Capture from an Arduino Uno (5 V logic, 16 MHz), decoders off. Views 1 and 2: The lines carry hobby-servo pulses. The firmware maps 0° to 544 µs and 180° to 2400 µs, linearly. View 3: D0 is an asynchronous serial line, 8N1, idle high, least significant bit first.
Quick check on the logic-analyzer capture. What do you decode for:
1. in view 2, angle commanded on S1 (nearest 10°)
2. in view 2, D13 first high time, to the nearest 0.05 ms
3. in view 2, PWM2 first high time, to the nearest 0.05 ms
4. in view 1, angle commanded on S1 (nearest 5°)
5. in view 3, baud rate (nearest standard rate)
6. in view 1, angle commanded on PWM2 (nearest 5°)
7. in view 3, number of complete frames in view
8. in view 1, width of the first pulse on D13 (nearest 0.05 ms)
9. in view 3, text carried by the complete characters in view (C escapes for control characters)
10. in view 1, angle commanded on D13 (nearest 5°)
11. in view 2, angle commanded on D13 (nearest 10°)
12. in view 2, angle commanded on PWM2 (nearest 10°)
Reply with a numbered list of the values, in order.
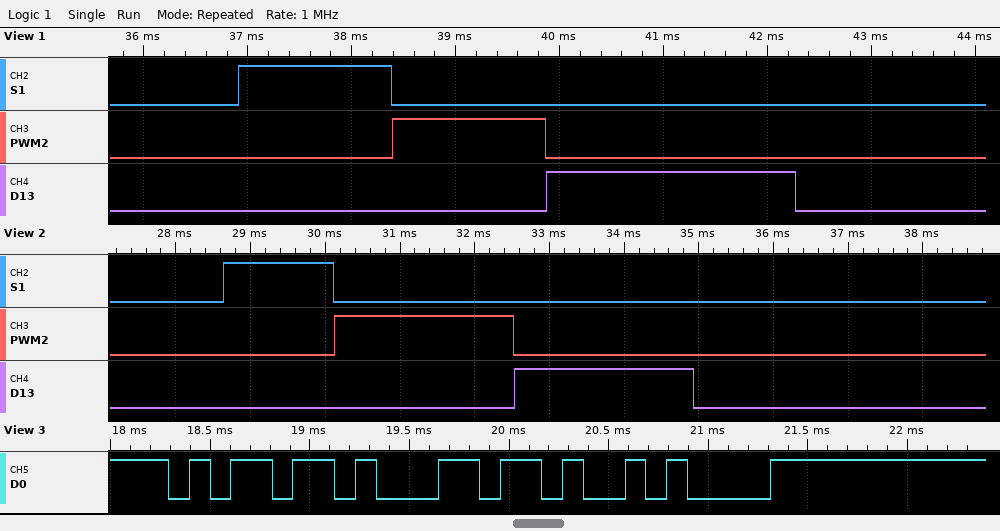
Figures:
1. 90°
2. 2.40 ms
3. 2.40 ms
4. 90°
5. 9600 baud
6. 90°
7. 3
8. 2.40 ms
9. "ml\n"
10. 180°
11. 180°
12. 180°
